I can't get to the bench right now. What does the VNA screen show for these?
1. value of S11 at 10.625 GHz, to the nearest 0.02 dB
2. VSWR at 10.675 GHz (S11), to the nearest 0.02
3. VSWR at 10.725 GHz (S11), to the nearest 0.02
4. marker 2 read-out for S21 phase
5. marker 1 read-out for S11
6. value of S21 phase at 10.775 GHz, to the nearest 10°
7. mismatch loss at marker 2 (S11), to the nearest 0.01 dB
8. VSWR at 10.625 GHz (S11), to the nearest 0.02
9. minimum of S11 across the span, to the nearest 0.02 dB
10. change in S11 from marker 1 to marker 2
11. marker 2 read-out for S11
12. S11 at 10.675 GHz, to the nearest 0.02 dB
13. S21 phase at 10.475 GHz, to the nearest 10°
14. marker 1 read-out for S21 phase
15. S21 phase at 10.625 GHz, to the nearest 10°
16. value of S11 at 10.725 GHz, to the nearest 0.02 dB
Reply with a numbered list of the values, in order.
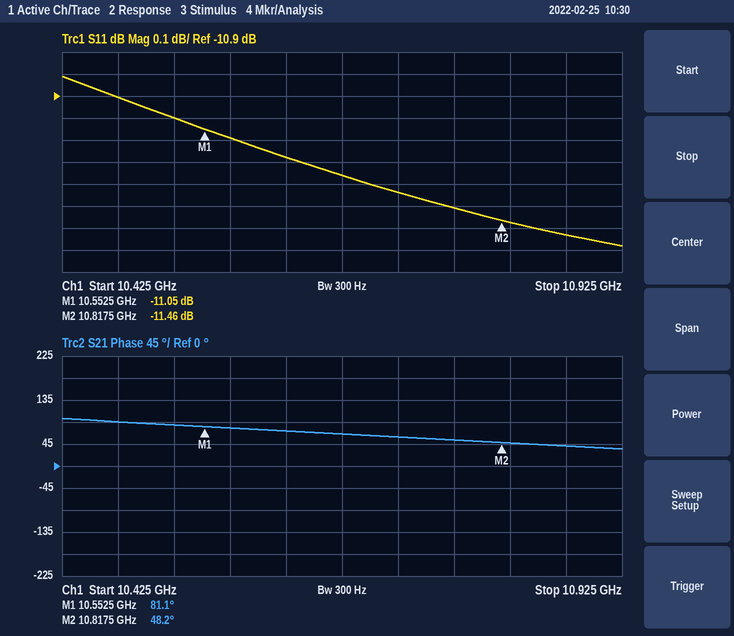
1. -11.18 dB
2. 1.76
3. 1.74
4. 48.2°
5. -11.05 dB
6. 50°
7. 0.32 dB
8. 1.76
9. -11.58 dB
10. -0.41 dB
11. -11.46 dB
12. -11.26 dB
13. 90°
14. 81.1°
15. 70°
16. -11.34 dB
